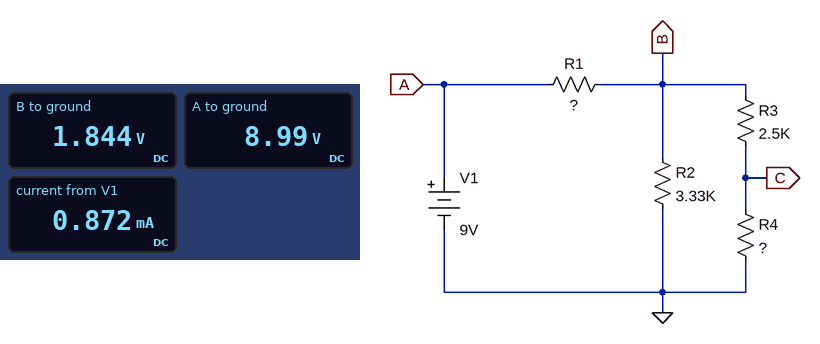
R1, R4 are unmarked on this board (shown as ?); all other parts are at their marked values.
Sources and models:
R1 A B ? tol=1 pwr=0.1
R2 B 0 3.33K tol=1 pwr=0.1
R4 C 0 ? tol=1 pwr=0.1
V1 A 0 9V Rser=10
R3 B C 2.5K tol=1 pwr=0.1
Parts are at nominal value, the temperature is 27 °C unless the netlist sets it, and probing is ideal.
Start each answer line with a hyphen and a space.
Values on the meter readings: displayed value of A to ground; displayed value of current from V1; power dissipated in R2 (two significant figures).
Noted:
- 8.99 V
- 0.872 mA
- 1.0 mW
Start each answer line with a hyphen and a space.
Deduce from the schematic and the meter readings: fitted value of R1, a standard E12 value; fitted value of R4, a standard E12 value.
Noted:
- 8.2 kΩ
- 3.3 kΩ
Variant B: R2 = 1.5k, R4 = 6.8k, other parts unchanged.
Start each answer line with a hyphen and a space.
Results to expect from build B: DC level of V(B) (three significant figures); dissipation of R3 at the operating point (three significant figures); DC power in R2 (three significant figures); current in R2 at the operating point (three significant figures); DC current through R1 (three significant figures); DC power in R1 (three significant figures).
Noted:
- 1.22 V
- 43.3 µW
- 998 µW
- 816 µA
- 947 µA
- 7.36 mW
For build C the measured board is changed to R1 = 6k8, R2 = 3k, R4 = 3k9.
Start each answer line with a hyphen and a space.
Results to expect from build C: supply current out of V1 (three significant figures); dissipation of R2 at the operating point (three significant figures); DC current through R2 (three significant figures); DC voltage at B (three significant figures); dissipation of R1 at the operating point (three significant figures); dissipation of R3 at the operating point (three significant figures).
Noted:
- 1.02 mA
- 1.44 mW
- 692 µA
- 2.08 V
- 7.03 mW
- 263 µW
